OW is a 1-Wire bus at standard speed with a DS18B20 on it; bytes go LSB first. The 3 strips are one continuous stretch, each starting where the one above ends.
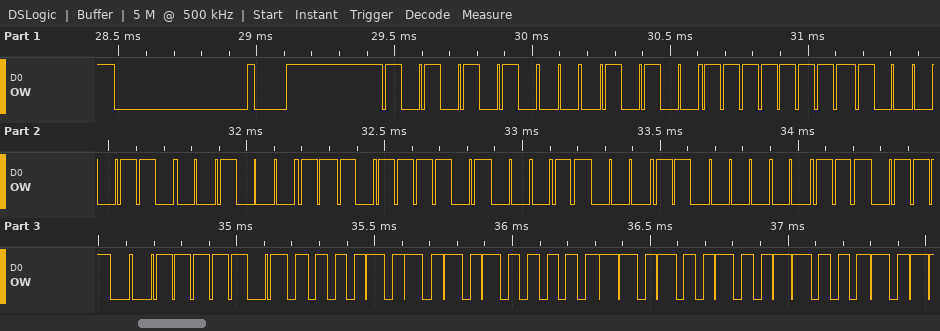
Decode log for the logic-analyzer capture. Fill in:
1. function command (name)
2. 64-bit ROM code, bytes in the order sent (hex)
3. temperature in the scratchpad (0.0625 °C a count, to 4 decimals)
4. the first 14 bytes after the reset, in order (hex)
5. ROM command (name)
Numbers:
Read Scratchpad
28 FF 61 C4 BD 18 03 77
85.0000 °C
55 28 FF 61 C4 BD 18 03 77 BE 50 05 4B 46
Match ROM
